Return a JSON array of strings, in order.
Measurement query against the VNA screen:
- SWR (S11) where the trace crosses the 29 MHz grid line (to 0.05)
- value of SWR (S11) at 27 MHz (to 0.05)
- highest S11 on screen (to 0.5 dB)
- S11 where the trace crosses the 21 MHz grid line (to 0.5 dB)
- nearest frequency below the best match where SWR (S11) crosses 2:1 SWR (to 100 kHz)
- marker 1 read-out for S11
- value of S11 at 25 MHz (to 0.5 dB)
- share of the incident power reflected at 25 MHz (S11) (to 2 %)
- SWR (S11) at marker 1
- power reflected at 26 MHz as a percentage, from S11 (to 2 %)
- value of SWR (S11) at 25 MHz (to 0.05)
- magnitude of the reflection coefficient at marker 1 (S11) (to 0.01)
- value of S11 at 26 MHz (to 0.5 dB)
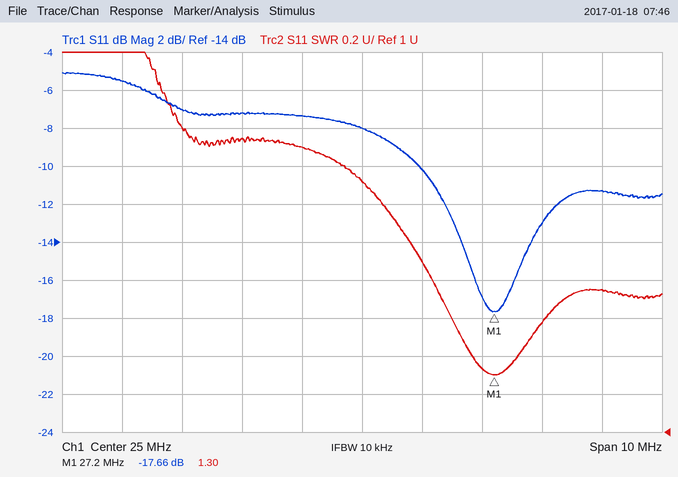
["1.75", "1.35", "-5.0 dB", "-5.5 dB", "25.8 MHz", "-17.66 dB", "-8.0 dB", "16 %", "1.30", "10 %", "2.30", "0.13", "-10.0 dB"]
